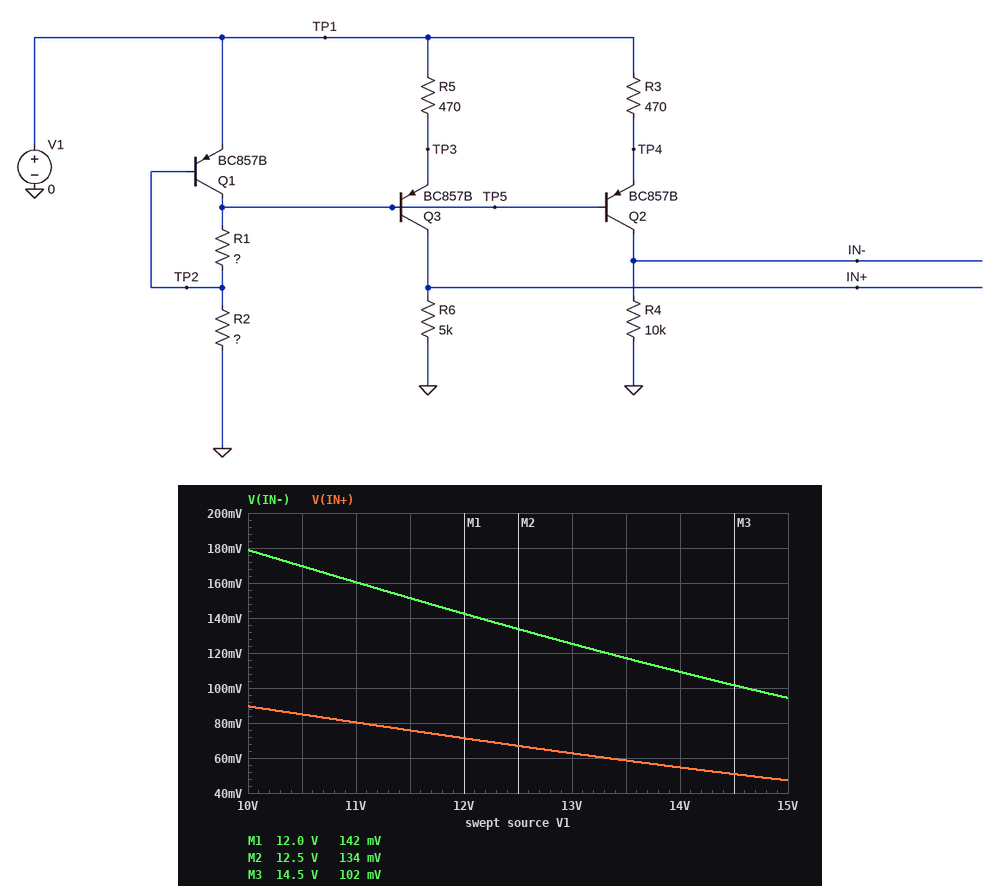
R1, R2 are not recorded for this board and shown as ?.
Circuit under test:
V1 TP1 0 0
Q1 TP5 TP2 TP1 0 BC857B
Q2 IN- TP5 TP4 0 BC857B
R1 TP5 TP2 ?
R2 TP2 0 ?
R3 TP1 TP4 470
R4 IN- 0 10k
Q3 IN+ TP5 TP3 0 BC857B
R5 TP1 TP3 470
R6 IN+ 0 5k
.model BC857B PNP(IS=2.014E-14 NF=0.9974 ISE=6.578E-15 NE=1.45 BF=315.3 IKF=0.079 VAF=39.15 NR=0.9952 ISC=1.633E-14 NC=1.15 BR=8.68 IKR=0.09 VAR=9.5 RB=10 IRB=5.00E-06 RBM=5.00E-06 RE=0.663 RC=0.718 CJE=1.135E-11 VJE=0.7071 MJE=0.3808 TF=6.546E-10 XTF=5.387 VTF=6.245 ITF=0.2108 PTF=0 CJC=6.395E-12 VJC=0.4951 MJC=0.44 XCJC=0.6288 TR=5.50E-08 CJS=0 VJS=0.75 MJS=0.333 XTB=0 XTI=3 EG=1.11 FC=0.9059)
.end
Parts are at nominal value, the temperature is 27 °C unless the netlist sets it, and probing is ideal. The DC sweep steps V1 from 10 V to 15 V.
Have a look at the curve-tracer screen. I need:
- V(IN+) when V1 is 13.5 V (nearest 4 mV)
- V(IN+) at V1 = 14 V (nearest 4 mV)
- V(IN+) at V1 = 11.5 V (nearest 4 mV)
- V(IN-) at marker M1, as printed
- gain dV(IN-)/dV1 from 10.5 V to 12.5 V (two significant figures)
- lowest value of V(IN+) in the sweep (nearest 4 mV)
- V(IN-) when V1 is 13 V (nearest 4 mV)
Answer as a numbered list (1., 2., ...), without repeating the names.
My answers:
1. 60 mV
2. 56 mV
3. 76 mV
4. 142 mV
5. -0.018 V/V
6. 48 mV
7. 124 mV
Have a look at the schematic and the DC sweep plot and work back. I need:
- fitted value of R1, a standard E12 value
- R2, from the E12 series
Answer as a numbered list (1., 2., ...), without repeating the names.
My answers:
1. 270 Ω
2. 39 kΩ
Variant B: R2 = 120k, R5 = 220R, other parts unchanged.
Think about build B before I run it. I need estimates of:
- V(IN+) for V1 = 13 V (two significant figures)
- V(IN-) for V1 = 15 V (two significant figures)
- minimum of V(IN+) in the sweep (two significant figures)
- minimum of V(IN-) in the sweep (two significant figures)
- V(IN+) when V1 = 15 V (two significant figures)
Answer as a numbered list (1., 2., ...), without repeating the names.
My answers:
1. 170 mV
2. 280 mV
3. 160 mV
4. 270 mV
5. 180 mV
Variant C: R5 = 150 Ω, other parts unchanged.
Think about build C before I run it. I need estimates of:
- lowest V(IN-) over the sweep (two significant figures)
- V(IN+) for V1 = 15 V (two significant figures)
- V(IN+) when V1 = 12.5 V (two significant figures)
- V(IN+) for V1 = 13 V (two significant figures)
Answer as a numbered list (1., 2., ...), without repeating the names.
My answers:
1. 94 mV
2. 53 mV
3. 78 mV
4. 72 mV
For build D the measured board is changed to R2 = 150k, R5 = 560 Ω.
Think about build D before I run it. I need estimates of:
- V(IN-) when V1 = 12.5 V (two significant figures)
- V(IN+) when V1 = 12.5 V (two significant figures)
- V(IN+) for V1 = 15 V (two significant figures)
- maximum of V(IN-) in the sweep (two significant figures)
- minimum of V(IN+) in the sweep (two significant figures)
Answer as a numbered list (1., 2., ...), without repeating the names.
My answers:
1. 280 mV
2. 130 mV
3. 140 mV
4. 290 mV
5. 120 mV
